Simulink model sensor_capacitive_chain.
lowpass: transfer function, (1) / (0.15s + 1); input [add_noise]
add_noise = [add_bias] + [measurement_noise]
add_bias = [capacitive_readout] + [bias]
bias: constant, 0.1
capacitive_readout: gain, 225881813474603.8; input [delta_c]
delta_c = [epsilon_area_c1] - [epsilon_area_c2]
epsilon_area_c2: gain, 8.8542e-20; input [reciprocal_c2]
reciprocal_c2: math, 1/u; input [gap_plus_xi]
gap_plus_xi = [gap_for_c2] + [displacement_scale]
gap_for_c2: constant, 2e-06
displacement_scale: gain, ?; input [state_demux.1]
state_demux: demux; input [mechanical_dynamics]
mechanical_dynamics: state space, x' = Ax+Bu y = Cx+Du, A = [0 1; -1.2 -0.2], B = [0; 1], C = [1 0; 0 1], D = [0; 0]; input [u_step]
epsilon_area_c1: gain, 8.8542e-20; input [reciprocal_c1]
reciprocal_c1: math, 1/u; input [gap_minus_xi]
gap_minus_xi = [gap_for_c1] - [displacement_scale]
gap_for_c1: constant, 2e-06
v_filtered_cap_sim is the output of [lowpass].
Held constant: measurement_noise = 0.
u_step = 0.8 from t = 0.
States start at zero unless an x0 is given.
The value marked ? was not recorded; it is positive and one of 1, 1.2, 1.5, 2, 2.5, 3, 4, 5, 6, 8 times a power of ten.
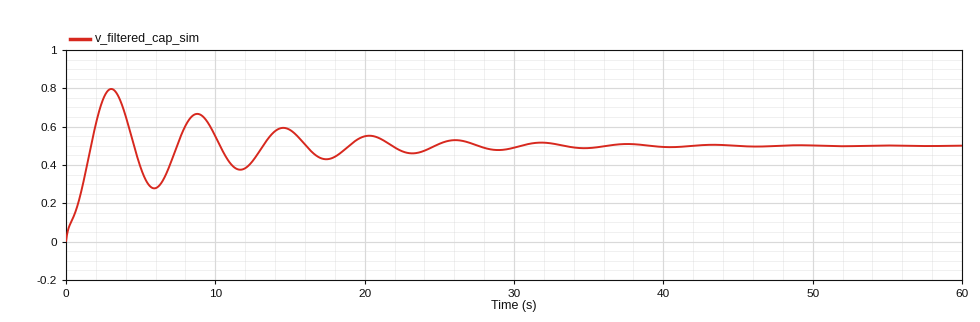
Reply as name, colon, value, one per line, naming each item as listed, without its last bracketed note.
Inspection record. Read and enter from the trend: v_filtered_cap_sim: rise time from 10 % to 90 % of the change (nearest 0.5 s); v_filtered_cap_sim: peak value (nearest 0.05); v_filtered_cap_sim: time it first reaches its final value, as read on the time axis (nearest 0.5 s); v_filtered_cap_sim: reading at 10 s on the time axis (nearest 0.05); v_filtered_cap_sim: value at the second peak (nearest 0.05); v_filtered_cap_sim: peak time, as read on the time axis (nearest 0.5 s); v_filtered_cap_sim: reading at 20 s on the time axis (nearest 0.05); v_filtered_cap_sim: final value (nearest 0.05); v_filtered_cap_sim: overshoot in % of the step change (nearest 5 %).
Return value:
v_filtered_cap_sim: rise time from 10 % to 90 % of the change: 1.5 s
v_filtered_cap_sim: peak value: 0.80
v_filtered_cap_sim: time it first reaches its final value, as read on the time axis: 1.5 s
v_filtered_cap_sim: reading at 10 s on the time axis: 0.55
v_filtered_cap_sim: value at the second peak: 0.65
v_filtered_cap_sim: peak time, as read on the time axis: 3.0 s
v_filtered_cap_sim: reading at 20 s on the time axis: 0.55
v_filtered_cap_sim: final value: 0.50
v_filtered_cap_sim: overshoot in % of the step change: 60 %
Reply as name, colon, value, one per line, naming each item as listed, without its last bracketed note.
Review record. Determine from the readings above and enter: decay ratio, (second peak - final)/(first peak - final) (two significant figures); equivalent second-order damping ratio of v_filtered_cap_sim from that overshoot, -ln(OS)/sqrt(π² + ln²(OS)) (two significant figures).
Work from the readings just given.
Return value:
decay ratio, (second peak - final)/(first peak - final): 0.50
equivalent second-order damping ratio of v_filtered_cap_sim from that overshoot, -ln(OS)/sqrt(π² + ln²(OS)): 0.16
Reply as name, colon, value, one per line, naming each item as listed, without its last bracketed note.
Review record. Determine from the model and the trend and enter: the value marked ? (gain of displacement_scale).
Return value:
the value marked ?: 6e-08
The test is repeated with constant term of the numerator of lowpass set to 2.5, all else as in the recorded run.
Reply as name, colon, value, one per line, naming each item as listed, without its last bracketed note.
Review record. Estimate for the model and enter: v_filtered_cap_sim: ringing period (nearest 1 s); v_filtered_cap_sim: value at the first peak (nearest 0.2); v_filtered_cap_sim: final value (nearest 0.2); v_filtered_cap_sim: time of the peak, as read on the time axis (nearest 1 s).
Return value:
v_filtered_cap_sim: ringing period: 6 s
v_filtered_cap_sim: value at the first peak: 2.0
v_filtered_cap_sim: final value: 1.2
v_filtered_cap_sim: time of the peak, as read on the time axis: 3 s
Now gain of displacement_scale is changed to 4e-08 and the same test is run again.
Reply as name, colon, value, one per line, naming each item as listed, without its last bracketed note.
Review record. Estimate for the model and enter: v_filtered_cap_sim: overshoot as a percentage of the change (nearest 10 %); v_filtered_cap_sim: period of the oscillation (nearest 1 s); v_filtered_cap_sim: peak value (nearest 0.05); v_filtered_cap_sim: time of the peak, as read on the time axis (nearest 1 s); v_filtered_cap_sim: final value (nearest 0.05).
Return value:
v_filtered_cap_sim: overshoot as a percentage of the change: 50 %
v_filtered_cap_sim: period of the oscillation: 6 s
v_filtered_cap_sim: peak value: 0.55
v_filtered_cap_sim: time of the peak, as read on the time axis: 3 s
v_filtered_cap_sim: final value: 0.35
